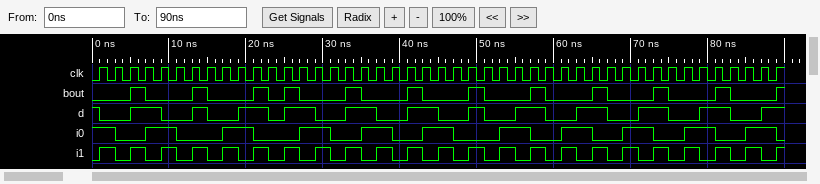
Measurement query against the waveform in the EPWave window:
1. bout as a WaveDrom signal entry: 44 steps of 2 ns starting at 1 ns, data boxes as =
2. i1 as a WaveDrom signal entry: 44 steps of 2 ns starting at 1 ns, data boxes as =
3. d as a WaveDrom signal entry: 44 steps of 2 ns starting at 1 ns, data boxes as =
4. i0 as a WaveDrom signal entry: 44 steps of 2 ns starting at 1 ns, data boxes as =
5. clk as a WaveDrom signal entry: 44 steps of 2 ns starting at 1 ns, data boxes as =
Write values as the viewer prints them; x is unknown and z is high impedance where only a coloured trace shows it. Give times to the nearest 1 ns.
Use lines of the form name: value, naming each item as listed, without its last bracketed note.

bout as a WaveDrom signal entry: 44 steps of 2 ns starting at 1 ns, data boxes as =: {name: 'bout', wave: '0.10..10..1010..10..10..10..10..10..10..10..'}
i1 as a WaveDrom signal entry: 44 steps of 2 ns starting at 1 ns, data boxes as =: {name: 'i1', wave: '10101010101010101010101010101010101010101010'}
d as a WaveDrom signal entry: 44 steps of 2 ns starting at 1 ns, data boxes as =: {name: 'd', wave: '0.1.0.10.1.01.0.1.0.1.0.10.1.0.1.0.1.0.1.0.1'}
i0 as a WaveDrom signal entry: 44 steps of 2 ns starting at 1 ns, data boxes as =: {name: 'i0', wave: '10.1.0..1.0..1.0.1.0.1.0..1.0.1.0.1.0.1.0.1.'}
clk as a WaveDrom signal entry: 44 steps of 2 ns starting at 1 ns, data boxes as =: {name: 'clk', wave: 'p...........................................'}
